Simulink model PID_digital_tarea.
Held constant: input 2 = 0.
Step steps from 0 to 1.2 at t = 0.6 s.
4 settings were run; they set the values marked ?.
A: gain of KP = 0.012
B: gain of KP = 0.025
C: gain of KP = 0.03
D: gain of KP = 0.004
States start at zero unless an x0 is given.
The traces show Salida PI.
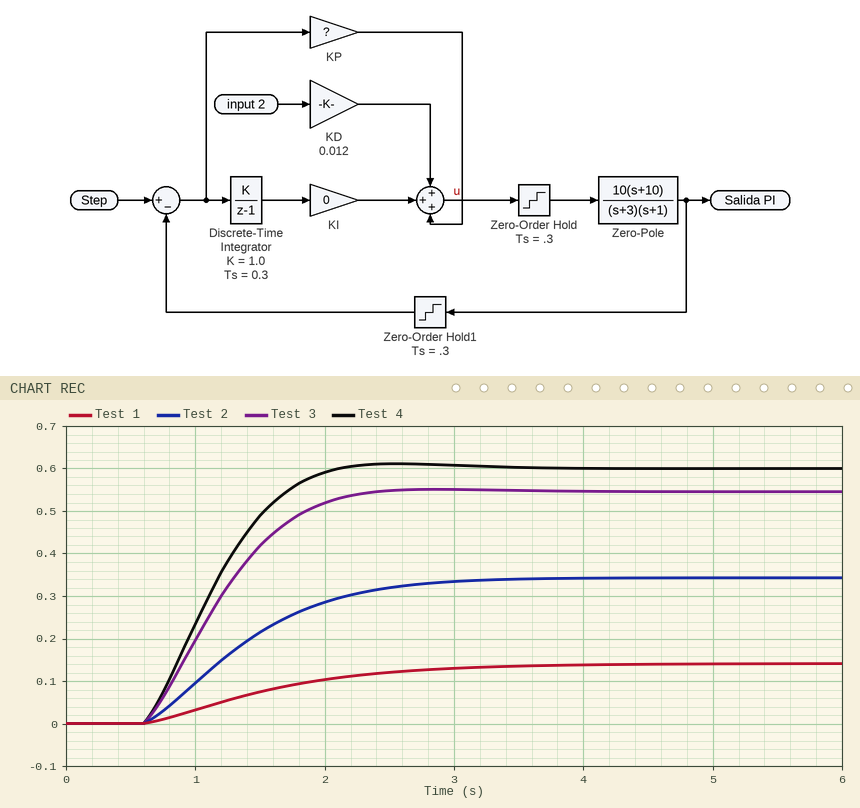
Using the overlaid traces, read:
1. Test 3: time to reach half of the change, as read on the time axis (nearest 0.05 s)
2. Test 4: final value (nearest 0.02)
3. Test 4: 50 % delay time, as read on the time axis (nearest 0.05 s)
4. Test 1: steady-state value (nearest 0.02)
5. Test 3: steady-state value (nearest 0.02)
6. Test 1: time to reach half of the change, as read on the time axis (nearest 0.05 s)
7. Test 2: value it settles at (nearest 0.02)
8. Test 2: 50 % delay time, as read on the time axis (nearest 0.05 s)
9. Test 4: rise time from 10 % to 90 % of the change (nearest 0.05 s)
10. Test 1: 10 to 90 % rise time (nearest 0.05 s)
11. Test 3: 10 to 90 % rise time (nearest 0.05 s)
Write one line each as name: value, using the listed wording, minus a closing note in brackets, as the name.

Test 3: time to reach half of the change, as read on the time axis: 1.15 s
Test 4: final value: 0.60
Test 4: 50 % delay time, as read on the time axis: 1.10 s
Test 1: steady-state value: 0.14
Test 3: steady-state value: 0.54
Test 1: time to reach half of the change, as read on the time axis: 1.45 s
Test 2: value it settles at: 0.34
Test 2: 50 % delay time, as read on the time axis: 1.30 s
Test 4: rise time from 10 % to 90 % of the change: 0.95 s
Test 1: 10 to 90 % rise time: 2.00 s
Test 3: 10 to 90 % rise time: 1.05 s
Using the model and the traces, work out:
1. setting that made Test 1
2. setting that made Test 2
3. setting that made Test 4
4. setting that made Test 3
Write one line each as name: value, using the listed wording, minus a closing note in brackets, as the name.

setting that made Test 1: D
setting that made Test 2: A
setting that made Test 4: C
setting that made Test 3: B
